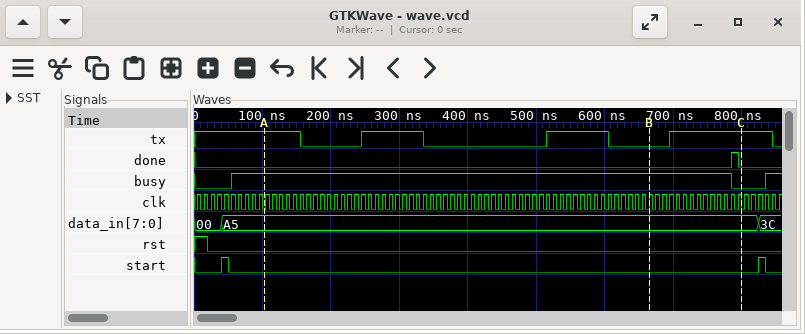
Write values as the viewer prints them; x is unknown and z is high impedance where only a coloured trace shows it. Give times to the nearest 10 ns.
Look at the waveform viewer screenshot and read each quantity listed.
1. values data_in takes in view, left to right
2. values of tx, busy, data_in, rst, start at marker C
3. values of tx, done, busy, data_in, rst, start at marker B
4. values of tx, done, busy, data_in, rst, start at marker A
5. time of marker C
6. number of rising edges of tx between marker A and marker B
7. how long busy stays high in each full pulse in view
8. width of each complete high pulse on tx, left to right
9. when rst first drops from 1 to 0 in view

00, A5, 3C
tx=1, busy=0, data_in=A5, rst=0, start=0
tx=0, done=0, busy=1, data_in=A5, rst=0, start=0
tx=1, done=0, busy=1, data_in=A5, rst=0, start=0
800 ns
2
730 ns
90 ns, 90 ns, 150 ns
20 ns
